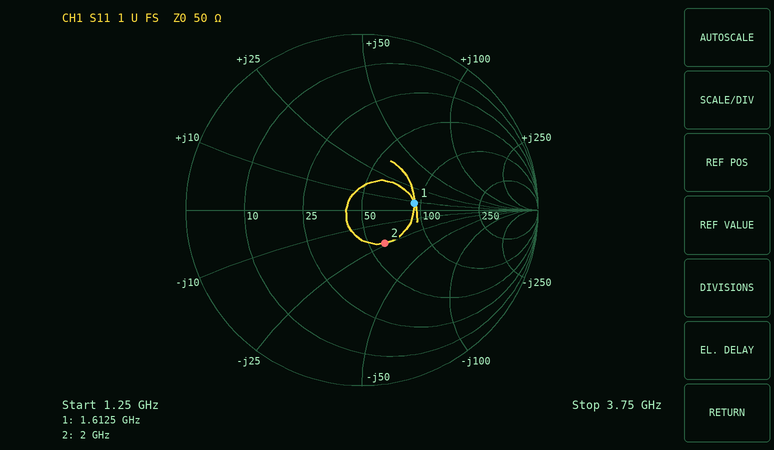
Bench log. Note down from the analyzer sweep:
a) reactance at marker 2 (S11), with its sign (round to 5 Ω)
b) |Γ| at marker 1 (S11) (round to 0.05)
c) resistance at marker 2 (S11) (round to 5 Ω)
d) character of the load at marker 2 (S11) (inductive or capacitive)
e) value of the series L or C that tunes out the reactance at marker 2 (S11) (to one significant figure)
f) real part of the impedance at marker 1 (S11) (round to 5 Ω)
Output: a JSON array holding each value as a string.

["-25 Ω", "0.30", "60 Ω", "capacitive", "2 nH", "90 Ω"]
